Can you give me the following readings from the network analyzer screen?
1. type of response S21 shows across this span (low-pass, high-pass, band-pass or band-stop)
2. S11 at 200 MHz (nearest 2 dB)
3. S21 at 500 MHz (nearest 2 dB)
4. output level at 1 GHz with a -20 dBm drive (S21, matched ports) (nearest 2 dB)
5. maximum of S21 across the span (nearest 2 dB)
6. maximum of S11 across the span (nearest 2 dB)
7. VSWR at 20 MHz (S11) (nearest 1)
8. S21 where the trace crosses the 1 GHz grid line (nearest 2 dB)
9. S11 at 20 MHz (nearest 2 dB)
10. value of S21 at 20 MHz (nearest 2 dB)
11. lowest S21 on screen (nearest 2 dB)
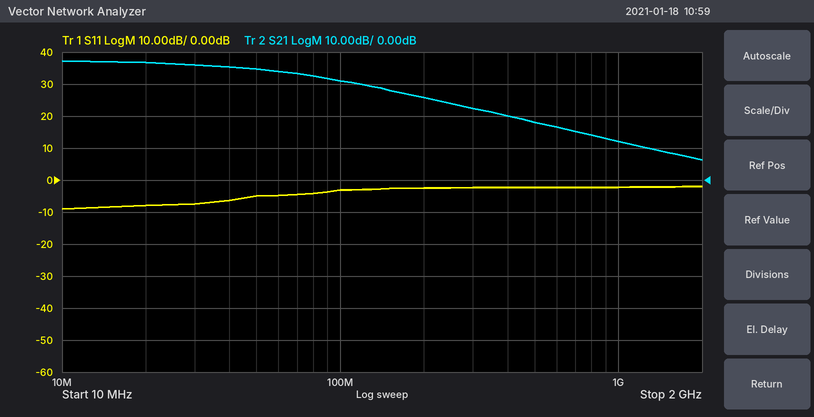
low-pass
-2 dB
18 dB
-8 dBm
38 dB
-2 dB
2
12 dB
-8 dB
36 dB
6 dB
